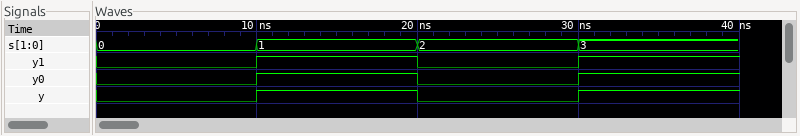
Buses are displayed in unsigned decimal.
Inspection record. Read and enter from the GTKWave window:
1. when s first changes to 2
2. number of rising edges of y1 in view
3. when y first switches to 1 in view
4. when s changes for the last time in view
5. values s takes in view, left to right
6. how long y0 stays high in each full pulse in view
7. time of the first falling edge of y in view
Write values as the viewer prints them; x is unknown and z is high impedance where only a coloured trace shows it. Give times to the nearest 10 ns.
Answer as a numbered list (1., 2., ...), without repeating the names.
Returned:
1. 20 ns
2. 2
3. 10 ns
4. 30 ns
5. 0, 1, 2, 3
6. 10 ns
7. 20 ns
